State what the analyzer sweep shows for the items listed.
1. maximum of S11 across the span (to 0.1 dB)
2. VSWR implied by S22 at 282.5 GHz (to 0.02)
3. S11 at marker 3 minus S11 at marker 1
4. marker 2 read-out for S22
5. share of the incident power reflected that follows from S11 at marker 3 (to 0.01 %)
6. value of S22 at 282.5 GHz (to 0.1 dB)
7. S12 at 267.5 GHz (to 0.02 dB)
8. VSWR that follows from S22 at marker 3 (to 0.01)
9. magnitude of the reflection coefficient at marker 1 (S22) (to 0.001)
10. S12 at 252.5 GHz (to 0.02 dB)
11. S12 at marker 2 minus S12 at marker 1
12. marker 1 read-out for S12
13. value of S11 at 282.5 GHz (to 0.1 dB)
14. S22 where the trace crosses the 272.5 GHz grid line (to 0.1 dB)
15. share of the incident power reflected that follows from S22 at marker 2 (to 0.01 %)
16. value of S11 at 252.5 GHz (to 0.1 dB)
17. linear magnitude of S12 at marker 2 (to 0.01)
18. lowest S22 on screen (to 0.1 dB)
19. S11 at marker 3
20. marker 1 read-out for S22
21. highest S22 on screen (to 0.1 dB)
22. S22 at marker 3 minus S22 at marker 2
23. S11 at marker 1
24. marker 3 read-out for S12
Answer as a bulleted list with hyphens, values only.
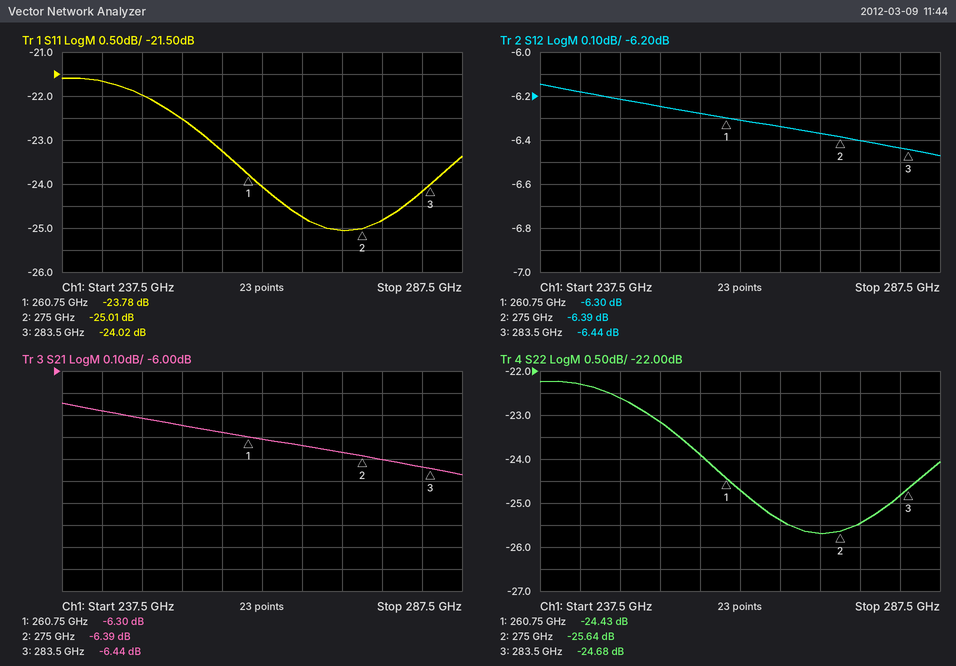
- -21.6 dB
- 1.12
- -0.24 dB
- -25.64 dB
- 0.40 %
- -24.8 dB
- -6.34 dB
- 1.12
- 0.060
- -6.24 dB
- -0.09 dB
- -6.30 dB
- -24.2 dB
- -25.7 dB
- 0.27 %
- -22.5 dB
- 0.48
- -25.7 dB
- -24.02 dB
- -24.43 dB
- -22.2 dB
- 0.96 dB
- -23.78 dB
- -6.44 dB
